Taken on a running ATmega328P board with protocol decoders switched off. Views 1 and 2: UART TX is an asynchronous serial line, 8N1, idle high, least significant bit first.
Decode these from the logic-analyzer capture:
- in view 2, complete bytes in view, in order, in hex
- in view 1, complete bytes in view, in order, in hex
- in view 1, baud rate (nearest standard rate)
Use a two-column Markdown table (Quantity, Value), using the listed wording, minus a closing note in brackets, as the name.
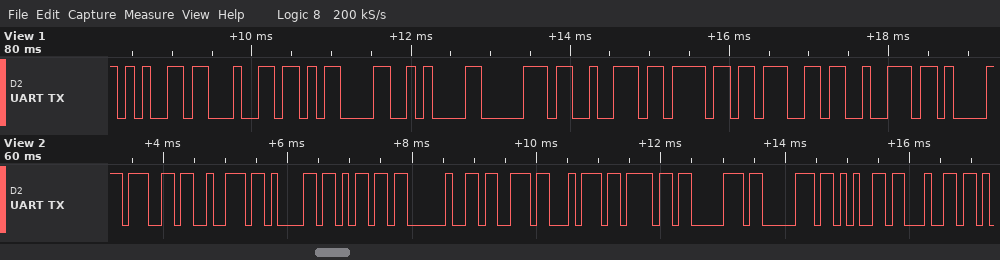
| Quantity | Value |
|---|---|
| in view 2, complete bytes in view, in order, in hex | 67 72 61 6D 20 73 74 6F 70 70 65 64 |
| in view 1, complete bytes in view, in order, in hex | 0x65 0x64 0x0D 0x0A 0x70 0x72 0x6F 0x67 0x72 |
| in view 1, baud rate | 9600 baud |
